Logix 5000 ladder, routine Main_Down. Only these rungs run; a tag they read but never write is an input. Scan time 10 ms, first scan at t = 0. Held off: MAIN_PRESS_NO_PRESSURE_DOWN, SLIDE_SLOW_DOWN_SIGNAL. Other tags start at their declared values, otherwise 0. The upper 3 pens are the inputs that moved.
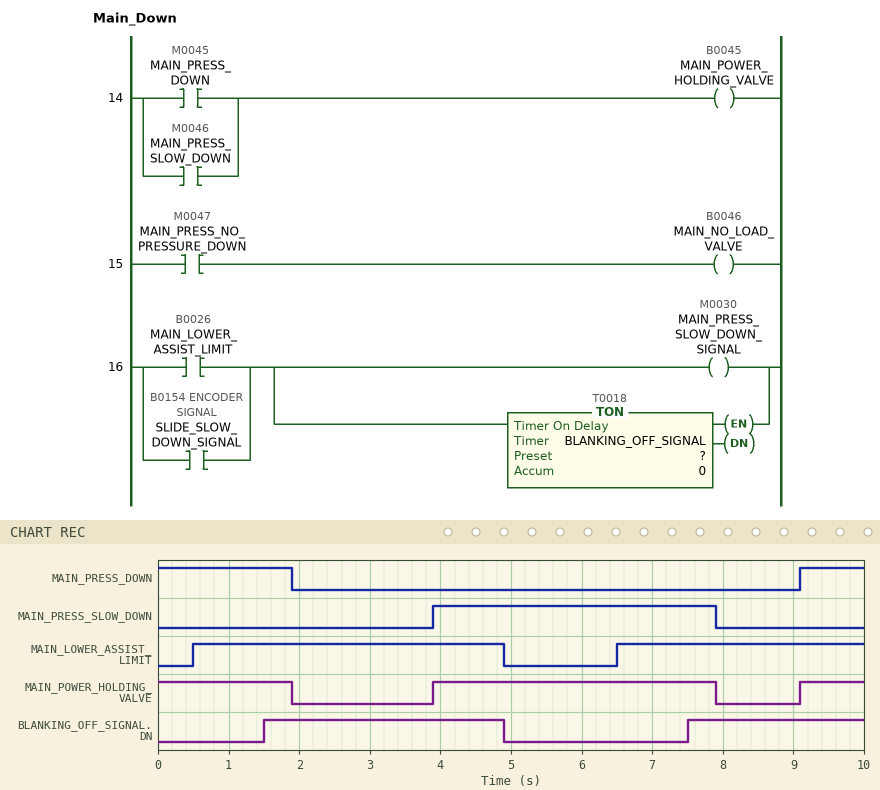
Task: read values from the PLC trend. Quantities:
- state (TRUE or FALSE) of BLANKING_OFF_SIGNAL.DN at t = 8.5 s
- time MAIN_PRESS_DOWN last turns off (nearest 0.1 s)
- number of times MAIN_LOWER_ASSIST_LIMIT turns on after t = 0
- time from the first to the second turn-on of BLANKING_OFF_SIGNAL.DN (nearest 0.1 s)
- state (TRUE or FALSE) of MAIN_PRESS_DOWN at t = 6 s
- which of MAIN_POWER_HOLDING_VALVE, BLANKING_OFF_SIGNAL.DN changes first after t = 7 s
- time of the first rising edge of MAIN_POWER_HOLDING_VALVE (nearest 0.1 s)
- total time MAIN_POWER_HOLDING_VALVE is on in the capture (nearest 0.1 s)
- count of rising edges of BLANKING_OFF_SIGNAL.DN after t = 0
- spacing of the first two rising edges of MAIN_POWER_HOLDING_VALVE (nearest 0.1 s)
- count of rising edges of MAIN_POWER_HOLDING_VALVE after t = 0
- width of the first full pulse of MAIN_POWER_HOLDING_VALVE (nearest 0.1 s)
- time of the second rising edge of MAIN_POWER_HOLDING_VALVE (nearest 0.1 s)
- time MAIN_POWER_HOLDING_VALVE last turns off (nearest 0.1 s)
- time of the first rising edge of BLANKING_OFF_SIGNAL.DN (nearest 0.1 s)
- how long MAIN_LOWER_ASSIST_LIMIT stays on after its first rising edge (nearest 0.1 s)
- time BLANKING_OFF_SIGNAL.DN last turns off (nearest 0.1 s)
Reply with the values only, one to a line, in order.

TRUE
1.9 s
2
6.0 s
FALSE
BLANKING_OFF_SIGNAL.DN
3.9 s
6.8 s
2
5.2 s
2
4.0 s
9.1 s
7.9 s
1.5 s
4.4 s
4.9 s
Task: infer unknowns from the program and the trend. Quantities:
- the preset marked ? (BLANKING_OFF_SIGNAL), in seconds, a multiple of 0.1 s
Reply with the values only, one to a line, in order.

1.0 s
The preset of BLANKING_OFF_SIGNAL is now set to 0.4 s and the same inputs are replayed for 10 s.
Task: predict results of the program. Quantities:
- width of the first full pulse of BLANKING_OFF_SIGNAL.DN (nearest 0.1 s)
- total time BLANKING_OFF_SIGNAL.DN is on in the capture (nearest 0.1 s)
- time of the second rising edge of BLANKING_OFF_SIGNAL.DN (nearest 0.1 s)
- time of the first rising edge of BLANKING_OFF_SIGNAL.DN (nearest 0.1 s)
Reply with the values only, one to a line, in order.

4.0 s
7.1 s
6.9 s
0.9 s
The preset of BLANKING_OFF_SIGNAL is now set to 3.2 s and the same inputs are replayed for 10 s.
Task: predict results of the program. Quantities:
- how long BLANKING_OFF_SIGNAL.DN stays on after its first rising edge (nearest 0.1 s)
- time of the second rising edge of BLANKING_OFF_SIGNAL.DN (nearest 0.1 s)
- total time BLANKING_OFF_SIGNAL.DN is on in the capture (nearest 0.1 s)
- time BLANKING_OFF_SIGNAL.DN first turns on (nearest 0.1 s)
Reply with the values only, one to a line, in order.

1.2 s
9.7 s
1.5 s
3.7 s
